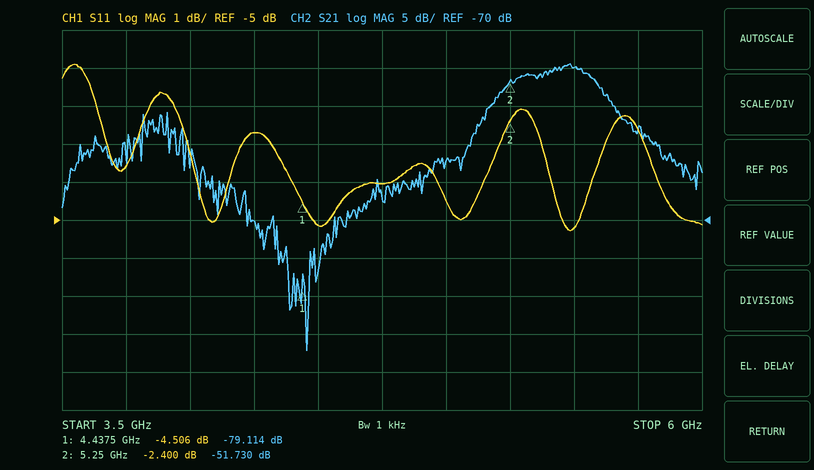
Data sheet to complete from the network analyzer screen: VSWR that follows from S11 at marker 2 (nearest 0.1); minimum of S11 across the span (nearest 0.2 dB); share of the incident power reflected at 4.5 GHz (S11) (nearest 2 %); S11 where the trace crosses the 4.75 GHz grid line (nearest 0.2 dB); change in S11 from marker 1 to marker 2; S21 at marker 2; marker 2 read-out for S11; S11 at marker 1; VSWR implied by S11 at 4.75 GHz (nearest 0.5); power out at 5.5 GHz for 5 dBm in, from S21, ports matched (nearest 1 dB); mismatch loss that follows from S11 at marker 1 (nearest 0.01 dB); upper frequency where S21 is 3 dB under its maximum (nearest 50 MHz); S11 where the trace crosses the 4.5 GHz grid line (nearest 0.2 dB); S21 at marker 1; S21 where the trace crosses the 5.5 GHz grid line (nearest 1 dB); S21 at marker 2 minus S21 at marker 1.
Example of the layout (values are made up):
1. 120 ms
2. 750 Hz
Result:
1. 7.3
2. -5.2 dB
3. 30 %
4. -4.0 dB
5. 2.106 dB
6. -51.730 dB
7. -2.400 dB
8. -4.506 dB
9. 4.5
10. -45 dBm
11. 1.90 dB
12. 5.60 GHz
13. -5.2 dB
14. -79.114 dB
15. -50 dB
16. 27.384 dB
